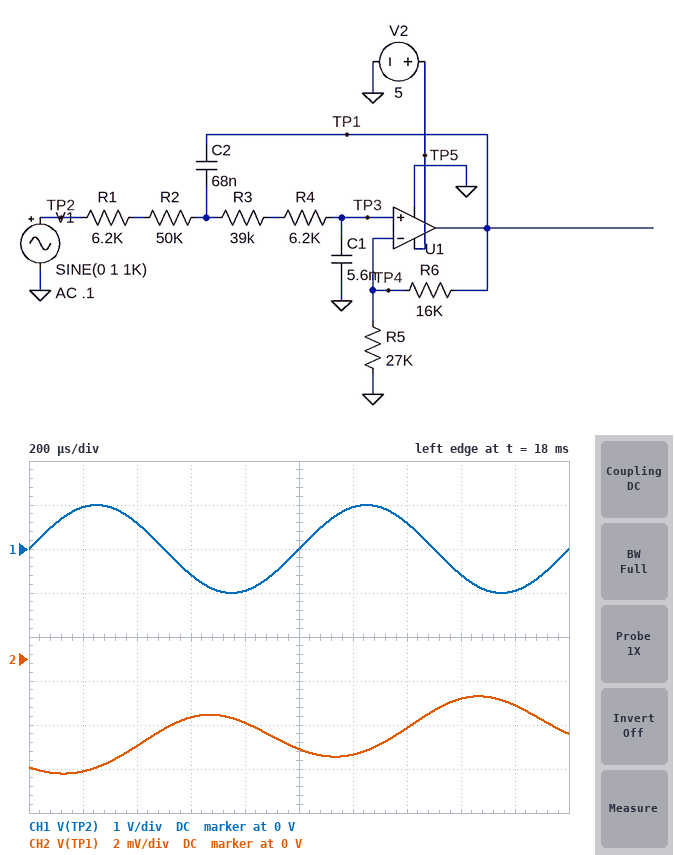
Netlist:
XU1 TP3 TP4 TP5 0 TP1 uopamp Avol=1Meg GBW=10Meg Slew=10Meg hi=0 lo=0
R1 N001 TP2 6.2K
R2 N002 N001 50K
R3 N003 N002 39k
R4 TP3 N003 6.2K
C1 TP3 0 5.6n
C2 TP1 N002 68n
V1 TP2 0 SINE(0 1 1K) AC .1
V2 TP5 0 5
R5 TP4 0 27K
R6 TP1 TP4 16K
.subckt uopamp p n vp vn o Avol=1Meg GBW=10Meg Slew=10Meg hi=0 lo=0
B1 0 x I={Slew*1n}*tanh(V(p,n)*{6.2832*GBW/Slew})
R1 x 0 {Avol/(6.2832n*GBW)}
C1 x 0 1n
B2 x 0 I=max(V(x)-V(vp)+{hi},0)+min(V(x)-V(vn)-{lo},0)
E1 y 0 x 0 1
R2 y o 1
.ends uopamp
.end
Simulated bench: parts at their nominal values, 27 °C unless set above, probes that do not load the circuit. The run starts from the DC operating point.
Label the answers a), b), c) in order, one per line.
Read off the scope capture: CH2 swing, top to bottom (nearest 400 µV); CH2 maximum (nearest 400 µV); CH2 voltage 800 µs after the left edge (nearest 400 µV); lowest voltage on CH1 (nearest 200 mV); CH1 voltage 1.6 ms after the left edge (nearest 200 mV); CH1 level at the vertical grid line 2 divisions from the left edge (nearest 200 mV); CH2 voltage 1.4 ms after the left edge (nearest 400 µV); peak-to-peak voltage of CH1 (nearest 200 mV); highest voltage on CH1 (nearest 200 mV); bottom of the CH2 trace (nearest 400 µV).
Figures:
a) 3.6 mV
b) -1.6 mV
c) -2.8 mV
d) -1.0 V
e) -600 mV
f) 600 mV
g) -3.2 mV
h) 2.0 V
i) 1.0 V
j) -5.2 mV
